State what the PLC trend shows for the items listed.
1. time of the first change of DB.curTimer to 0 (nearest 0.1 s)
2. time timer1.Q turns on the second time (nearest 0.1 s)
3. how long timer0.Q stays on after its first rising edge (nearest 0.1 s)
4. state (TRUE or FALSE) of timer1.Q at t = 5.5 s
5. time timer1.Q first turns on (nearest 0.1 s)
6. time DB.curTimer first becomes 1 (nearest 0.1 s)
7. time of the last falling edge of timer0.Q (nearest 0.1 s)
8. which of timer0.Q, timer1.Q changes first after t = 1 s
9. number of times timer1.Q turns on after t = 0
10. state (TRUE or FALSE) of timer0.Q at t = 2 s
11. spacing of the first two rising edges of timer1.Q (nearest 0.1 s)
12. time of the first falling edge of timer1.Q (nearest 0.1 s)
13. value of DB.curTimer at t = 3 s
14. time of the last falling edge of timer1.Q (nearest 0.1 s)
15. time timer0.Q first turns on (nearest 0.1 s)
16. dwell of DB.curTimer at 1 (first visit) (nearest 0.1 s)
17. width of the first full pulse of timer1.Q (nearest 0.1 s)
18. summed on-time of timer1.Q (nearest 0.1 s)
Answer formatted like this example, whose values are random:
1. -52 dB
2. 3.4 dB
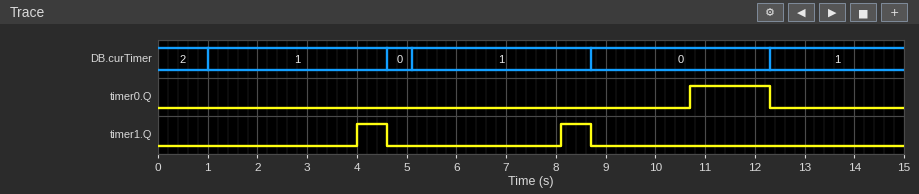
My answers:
1. 4.6 s
2. 8.1 s
3. 1.6 s
4. FALSE
5. 4.0 s
6. 1.0 s
7. 12.3 s
8. timer1.Q
9. 2
10. FALSE
11. 4.1 s
12. 4.6 s
13. 1
14. 8.7 s
15. 10.7 s
16. 3.6 s
17. 0.6 s
18. 1.2 s
